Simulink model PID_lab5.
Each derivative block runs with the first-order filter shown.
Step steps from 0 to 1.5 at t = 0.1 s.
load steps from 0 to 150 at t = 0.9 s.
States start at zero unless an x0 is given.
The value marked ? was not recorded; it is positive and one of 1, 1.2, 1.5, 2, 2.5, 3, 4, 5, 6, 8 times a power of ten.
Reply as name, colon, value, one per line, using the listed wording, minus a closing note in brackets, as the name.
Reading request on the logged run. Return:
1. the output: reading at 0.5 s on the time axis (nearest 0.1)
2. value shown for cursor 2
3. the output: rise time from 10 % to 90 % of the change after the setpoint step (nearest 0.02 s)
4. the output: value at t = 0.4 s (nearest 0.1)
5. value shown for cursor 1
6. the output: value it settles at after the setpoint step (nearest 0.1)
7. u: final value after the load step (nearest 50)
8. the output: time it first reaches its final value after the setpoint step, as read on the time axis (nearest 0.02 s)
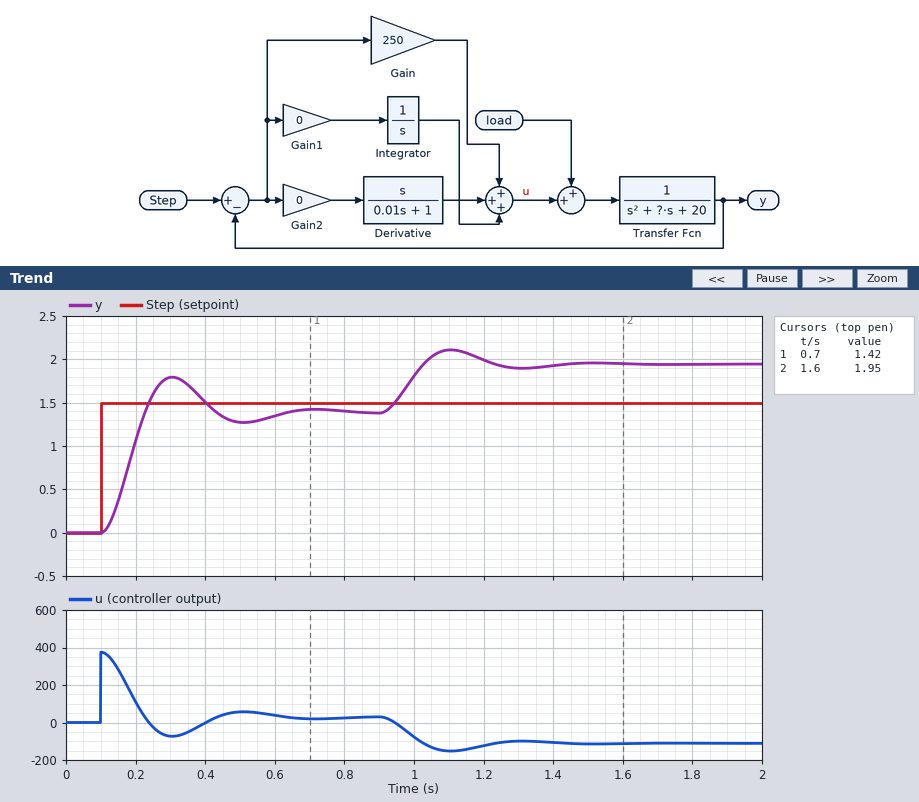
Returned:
the output: reading at 0.5 s on the time axis: 1.3
value shown for cursor 2: 1.95
the output: rise time from 10 % to 90 % of the change after the setpoint step: 0.08 s
the output: value at t = 0.4 s: 1.5
value shown for cursor 1: 1.42
the output: value it settles at after the setpoint step: 1.4
u: final value after the load step: -100
the output: time it first reaches its final value after the setpoint step, as read on the time axis: 0.22 s
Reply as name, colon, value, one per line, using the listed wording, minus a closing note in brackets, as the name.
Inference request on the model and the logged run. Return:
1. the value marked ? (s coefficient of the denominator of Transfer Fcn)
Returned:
the value marked ?: 12
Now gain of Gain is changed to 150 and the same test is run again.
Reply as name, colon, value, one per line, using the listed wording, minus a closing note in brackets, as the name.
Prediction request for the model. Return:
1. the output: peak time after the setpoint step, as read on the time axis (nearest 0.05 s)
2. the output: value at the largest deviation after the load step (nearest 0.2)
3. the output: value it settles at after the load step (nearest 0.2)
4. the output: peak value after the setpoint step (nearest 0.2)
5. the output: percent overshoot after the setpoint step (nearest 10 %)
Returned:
the output: peak time after the setpoint step, as read on the time axis: 0.35 s
the output: value at the largest deviation after the load step: 2.4
the output: value it settles at after the load step: 2.2
the output: peak value after the setpoint step: 1.6
the output: percent overshoot after the setpoint step: 20 %
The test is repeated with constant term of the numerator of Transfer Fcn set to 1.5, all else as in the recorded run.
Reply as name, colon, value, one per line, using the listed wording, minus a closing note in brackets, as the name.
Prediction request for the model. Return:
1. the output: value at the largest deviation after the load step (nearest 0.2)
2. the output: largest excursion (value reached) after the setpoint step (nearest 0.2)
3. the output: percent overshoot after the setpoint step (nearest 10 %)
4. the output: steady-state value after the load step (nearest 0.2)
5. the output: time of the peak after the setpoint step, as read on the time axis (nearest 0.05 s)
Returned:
the output: value at the largest deviation after the load step: 2.2
the output: largest excursion (value reached) after the setpoint step: 2.0
the output: percent overshoot after the setpoint step: 40 %
the output: steady-state value after the load step: 2.0
the output: time of the peak after the setpoint step, as read on the time axis: 0.25 s
